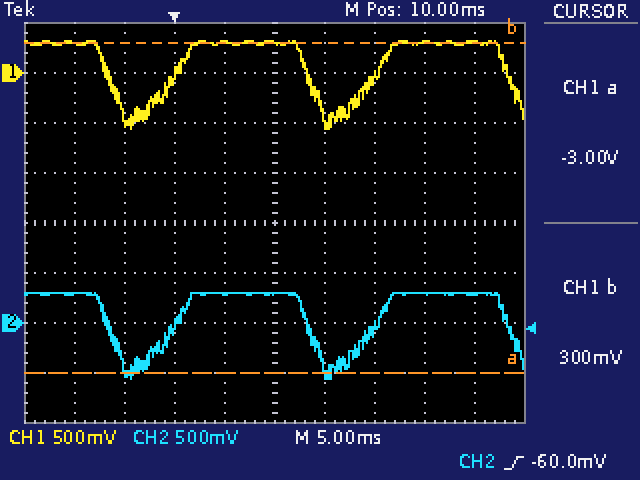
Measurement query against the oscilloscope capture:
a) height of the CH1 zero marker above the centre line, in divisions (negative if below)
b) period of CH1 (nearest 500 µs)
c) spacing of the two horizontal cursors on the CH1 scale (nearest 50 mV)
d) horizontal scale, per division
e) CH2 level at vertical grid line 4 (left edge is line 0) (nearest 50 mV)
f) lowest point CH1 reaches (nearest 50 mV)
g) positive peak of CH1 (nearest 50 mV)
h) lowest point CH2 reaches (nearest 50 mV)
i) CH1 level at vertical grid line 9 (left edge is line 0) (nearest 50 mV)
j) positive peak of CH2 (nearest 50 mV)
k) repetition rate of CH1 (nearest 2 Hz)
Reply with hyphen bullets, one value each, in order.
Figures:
- +3.0 div
- 20.0 ms
- 3.30 V
- 5 ms
- 300 mV
- -550 mV
- 300 mV
- -550 mV
- 300 mV
- 300 mV
- 50 Hz
